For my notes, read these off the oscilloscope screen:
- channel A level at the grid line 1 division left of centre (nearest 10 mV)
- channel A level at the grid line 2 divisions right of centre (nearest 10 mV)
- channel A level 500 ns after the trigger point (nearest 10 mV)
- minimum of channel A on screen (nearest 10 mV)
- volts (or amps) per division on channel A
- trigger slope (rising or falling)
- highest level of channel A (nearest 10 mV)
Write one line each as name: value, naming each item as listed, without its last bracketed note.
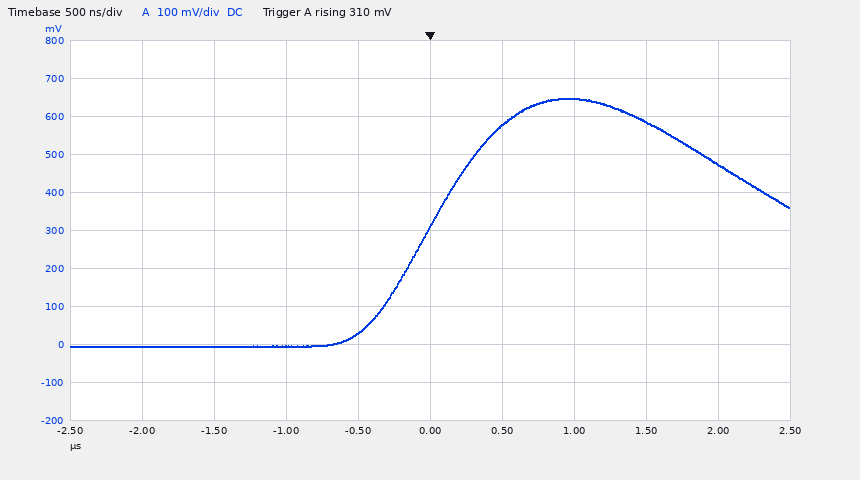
channel A level at the grid line 1 division left of centre: 30 mV
channel A level at the grid line 2 divisions right of centre: 650 mV
channel A level 500 ns after the trigger point: 580 mV
minimum of channel A on screen: -10 mV
volts (or amps) per division on channel A: 100 mV
trigger slope: rising
highest level of channel A: 650 mV
